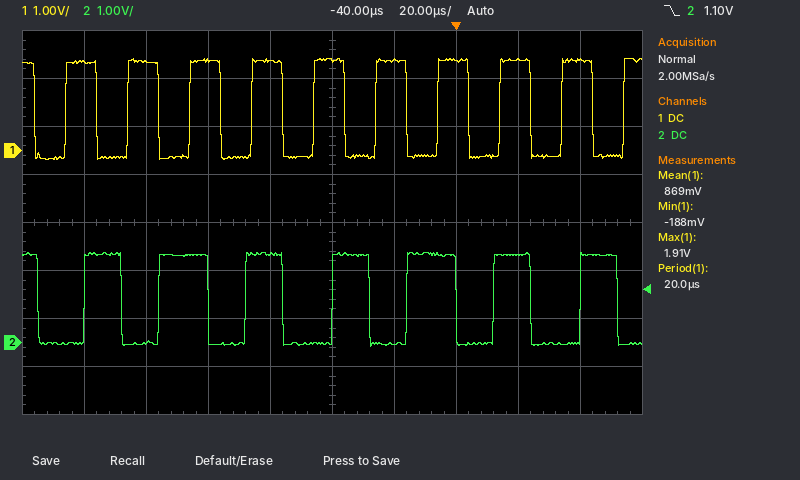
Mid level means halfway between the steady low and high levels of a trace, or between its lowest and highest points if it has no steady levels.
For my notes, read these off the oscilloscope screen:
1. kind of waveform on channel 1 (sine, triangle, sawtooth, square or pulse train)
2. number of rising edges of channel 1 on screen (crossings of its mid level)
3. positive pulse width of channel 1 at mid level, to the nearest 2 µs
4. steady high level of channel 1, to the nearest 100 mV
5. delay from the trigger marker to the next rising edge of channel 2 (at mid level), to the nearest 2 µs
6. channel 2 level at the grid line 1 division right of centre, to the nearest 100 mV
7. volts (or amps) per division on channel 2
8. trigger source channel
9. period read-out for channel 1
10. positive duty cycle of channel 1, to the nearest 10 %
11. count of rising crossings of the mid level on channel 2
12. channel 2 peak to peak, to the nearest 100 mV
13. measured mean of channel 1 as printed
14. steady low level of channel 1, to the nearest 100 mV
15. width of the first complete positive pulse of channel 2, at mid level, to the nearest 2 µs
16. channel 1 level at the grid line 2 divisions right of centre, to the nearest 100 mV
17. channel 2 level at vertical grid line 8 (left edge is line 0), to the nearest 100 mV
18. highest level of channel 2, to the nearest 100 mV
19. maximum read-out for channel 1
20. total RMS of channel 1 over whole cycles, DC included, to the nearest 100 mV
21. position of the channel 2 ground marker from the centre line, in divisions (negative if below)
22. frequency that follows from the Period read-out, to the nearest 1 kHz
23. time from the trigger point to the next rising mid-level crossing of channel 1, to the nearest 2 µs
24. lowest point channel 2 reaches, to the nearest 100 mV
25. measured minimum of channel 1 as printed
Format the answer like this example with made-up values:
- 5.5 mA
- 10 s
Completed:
- square
- 10
- 10 µs
- 1.9 V
- 12 µs
- 0.0 V
- 1 V
- channel 2
- 20.0 µs
- 50 %
- 7
- 2.0 V
- 869 mV
- -100 mV
- 12 µs
- 1.9 V
- 1.8 V
- 1.9 V
- 1.91 V
- 1.3 V
- -2.5 div
- 50 kHz
- 14 µs
- -100 mV
- -188 mV
